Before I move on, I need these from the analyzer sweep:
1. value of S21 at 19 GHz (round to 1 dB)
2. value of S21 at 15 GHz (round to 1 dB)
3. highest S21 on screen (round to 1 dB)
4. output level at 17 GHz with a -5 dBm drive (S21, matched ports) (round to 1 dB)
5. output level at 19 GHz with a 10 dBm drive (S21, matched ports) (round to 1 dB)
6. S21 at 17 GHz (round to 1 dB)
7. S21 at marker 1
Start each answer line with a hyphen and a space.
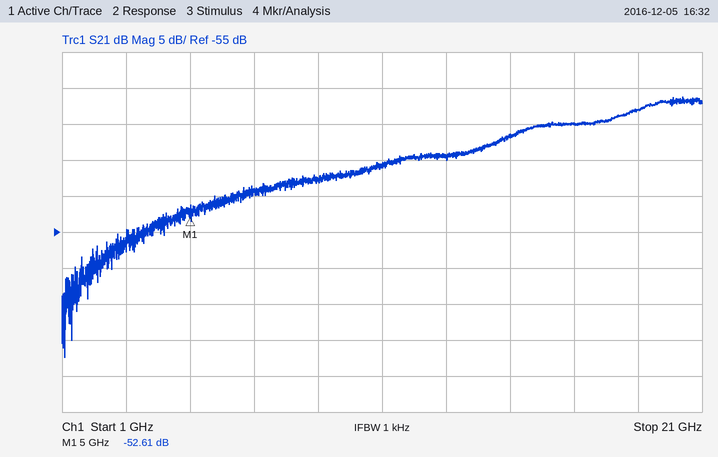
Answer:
- -38 dB
- -42 dB
- -36 dB
- -45 dBm
- -28 dBm
- -40 dB
- -52.61 dB
